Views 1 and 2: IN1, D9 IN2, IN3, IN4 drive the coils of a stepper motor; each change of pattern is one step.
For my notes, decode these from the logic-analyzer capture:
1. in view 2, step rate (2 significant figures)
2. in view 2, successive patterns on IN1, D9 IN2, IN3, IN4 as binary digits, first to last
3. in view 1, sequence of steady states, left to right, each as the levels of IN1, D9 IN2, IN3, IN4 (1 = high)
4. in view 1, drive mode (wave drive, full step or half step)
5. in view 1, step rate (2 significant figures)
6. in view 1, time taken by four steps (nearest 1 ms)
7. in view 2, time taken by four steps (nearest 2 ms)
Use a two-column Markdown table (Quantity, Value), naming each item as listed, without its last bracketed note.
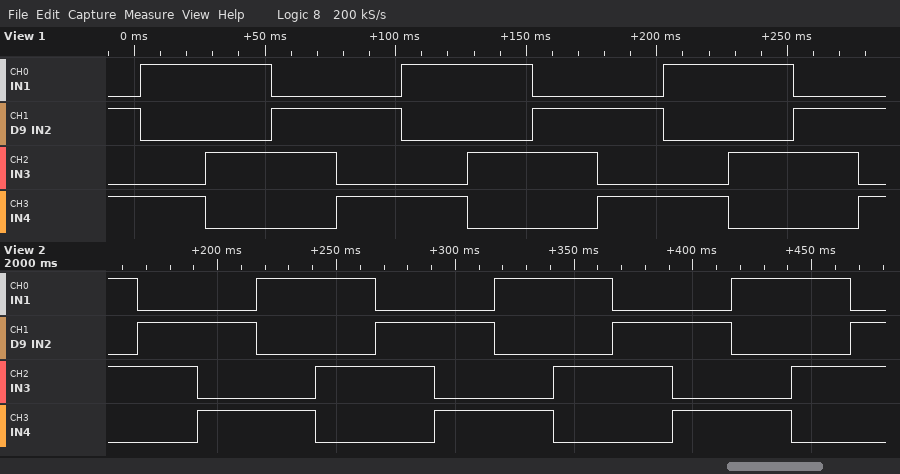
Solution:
| Quantity | Value |
|---|---|
| in view 2, step rate | 40 steps/s |
| in view 2, successive patterns on IN1, D9 IN2, IN3, IN4 as binary digits, first to last | 1010 0110 0101 1001 1010 0110 0101 1001 1010 0110 0101 1001 1010 0110 |
| in view 1, sequence of steady states, left to right, each as the levels of IN1, D9 IN2, IN3, IN4 | 0101 1001 1010 0110 0101 1001 1010 0110 0101 1001 1010 0110 0101 |
| in view 1, drive mode | full step |
| in view 1, step rate | 40 steps/s |
| in view 1, time taken by four steps | 100 ms |
| in view 2, time taken by four steps | 100 ms |
